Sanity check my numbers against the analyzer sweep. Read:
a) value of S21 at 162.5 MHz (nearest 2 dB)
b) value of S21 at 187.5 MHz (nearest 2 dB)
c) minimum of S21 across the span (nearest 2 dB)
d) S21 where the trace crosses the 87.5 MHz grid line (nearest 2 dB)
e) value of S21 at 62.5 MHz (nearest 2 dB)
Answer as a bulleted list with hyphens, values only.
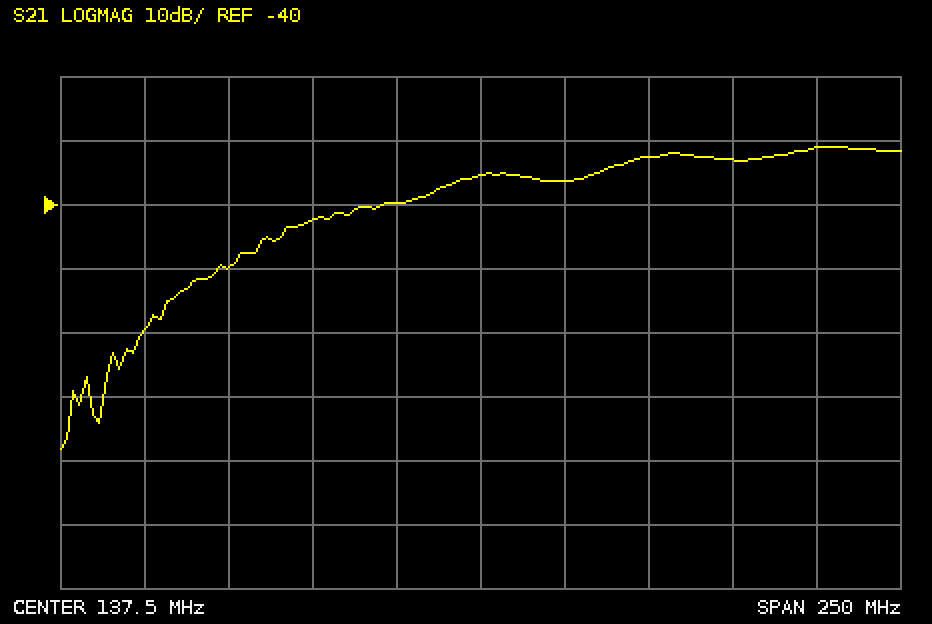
- -36 dB
- -32 dB
- -78 dB
- -42 dB
- -50 dB
